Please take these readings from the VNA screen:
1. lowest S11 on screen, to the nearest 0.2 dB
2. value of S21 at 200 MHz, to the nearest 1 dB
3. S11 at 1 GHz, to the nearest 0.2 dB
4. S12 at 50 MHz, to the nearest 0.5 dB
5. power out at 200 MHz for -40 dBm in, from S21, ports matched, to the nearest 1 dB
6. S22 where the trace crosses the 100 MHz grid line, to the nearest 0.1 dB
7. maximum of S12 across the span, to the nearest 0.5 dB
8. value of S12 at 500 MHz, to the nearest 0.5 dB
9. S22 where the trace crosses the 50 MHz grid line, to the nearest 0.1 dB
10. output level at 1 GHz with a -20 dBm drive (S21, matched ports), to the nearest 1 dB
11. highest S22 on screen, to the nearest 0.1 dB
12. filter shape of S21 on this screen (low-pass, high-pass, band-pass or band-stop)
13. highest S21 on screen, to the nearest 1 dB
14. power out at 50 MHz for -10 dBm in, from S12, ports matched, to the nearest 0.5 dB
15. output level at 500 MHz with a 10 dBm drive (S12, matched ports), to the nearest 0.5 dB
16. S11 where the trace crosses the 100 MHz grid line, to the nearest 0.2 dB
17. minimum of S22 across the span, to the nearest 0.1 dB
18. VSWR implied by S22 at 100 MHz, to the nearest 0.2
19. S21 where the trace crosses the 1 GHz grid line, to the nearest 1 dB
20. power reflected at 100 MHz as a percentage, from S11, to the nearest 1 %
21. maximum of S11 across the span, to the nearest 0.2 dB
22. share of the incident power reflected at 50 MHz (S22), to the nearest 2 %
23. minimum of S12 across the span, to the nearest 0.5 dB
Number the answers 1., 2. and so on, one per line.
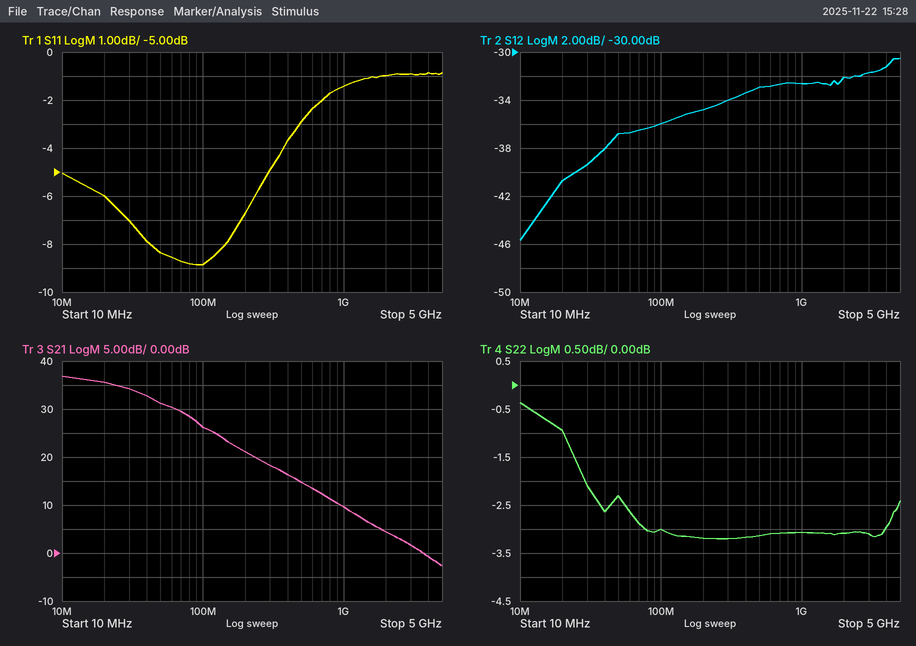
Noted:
1. -8.8 dB
2. 21 dB
3. -1.4 dB
4. -37.0 dB
5. -19 dBm
6. -3.0 dB
7. -30.5 dB
8. -33.0 dB
9. -2.3 dB
10. -10 dBm
11. -0.4 dB
12. low-pass
13. 37 dB
14. -47.0 dBm
15. -23.0 dBm
16. -8.8 dB
17. -3.2 dB
18. 5.8
19. 10 dB
20. 13 %
21. -0.8 dB
22. 58 %
23. -45.5 dB
